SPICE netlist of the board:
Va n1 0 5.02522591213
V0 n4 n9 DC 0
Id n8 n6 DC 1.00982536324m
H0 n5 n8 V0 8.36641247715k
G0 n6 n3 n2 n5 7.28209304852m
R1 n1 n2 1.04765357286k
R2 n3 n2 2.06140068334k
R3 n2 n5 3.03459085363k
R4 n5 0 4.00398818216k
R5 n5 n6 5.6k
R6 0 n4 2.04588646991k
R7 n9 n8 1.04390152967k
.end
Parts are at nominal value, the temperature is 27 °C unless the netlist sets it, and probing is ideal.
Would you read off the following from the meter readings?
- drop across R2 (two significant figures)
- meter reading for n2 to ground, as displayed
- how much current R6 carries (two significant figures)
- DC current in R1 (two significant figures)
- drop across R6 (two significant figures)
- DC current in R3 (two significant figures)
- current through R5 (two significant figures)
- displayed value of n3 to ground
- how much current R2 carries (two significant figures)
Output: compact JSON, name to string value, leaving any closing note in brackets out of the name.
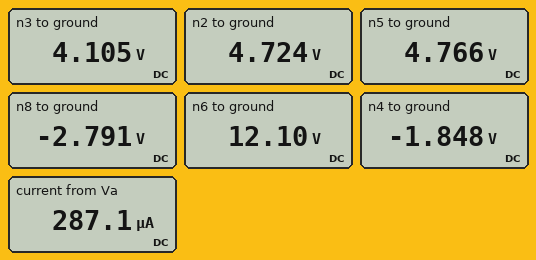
{"drop across R2": "620 mV", "meter reading for n2 to ground, as displayed": "4.724 V", "how much current R6 carries": "900 µA", "DC current in R1": "290 µA", "drop across R6": "1.8 V", "DC current in R3": "14 µA", "current through R5": "1.3 mA", "displayed value of n3 to ground": "4.105 V", "how much current R2 carries": "300 µA"}
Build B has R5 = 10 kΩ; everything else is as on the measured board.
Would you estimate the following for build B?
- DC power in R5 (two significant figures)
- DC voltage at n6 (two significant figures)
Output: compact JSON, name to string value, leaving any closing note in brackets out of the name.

{"DC power in R5": "17 mW", "DC voltage at n6": "18 V"}
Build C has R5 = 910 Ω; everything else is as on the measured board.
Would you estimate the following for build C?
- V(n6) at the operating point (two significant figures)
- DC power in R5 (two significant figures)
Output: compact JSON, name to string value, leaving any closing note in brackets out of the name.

{"V(n6) at the operating point": "6.0 V", "DC power in R5": "1.6 mW"}
